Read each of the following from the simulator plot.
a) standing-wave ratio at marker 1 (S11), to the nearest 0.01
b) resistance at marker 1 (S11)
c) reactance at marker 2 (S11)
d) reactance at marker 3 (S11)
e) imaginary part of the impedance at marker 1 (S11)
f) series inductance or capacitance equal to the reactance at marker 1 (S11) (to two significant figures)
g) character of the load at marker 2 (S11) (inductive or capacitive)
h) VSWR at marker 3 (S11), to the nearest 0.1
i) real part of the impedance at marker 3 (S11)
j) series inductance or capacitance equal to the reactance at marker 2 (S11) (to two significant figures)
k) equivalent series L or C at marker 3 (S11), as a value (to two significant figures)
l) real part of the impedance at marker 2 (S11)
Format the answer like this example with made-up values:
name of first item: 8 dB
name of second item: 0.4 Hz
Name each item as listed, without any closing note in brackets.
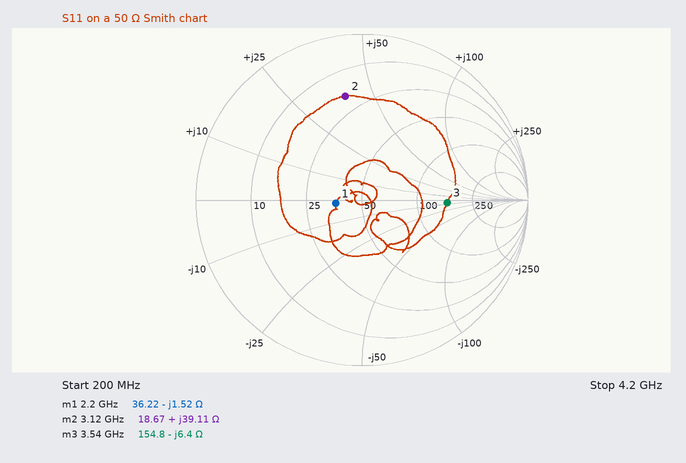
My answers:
standing-wave ratio at marker 1 (S11), to the nearest 0.01: 1.38
resistance at marker 1: 36.22 Ω
reactance at marker 2: +39.11 Ω
reactance at marker 3: -6.4 Ω
imaginary part of the impedance at marker 1: -1.52 Ω
series inductance or capacitance equal to the reactance at marker 1 (S11): 48 pF
character of the load at marker 2 (S11): inductive
VSWR at marker 3 (S11), to the nearest 0.1: 3.1
real part of the impedance at marker 3: 154.8 Ω
series inductance or capacitance equal to the reactance at marker 2 (S11): 2.0 nH
equivalent series L or C at marker 3 (S11), as a value: 7.0 pF
real part of the impedance at marker 2: 18.67 Ω
